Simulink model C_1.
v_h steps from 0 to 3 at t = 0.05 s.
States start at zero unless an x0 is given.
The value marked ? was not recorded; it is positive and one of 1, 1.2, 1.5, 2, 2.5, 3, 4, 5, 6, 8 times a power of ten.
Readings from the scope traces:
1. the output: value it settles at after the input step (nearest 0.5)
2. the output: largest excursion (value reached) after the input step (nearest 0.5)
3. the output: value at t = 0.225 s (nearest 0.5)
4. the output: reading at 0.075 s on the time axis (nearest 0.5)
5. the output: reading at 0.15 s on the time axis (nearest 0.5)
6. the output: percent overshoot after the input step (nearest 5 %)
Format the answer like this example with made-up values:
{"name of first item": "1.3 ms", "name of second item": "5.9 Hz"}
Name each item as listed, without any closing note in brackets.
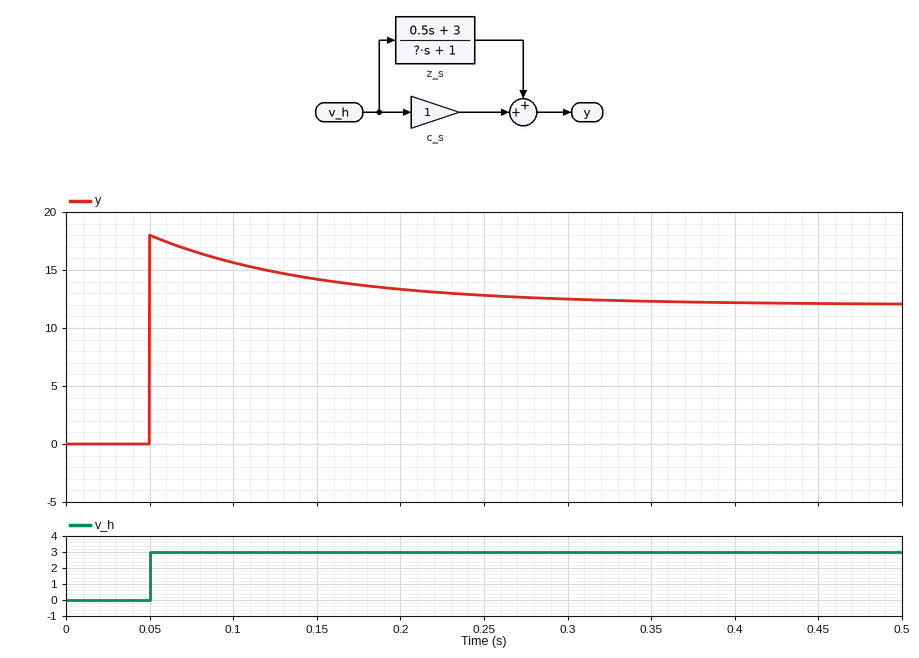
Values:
{"the output: value it settles at after the input step": "12.0", "the output: largest excursion (value reached) after the input step": "18.0", "the output: value at t = 0.225 s": "13.0", "the output: reading at 0.075 s on the time axis": "16.5", "the output: reading at 0.15 s on the time axis": "14.0", "the output: percent overshoot after the input step": "50 %"}
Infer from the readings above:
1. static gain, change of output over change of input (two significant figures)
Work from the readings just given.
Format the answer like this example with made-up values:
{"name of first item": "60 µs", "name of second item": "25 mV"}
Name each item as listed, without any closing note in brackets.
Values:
{"static gain, change of output over change of input": "4.0"}
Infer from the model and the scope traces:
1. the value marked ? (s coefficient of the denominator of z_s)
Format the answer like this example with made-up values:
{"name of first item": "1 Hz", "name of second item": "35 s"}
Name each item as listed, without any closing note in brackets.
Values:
{"the value marked ?": "0.1"}
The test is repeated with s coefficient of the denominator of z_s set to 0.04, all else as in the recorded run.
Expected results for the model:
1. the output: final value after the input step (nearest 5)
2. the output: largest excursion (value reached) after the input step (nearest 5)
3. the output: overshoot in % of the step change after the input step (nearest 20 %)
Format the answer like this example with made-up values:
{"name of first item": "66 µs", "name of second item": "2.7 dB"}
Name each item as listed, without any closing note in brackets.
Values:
{"the output: final value after the input step": "10", "the output: largest excursion (value reached) after the input step": "40", "the output: overshoot in % of the step change after the input step": "240 %"}
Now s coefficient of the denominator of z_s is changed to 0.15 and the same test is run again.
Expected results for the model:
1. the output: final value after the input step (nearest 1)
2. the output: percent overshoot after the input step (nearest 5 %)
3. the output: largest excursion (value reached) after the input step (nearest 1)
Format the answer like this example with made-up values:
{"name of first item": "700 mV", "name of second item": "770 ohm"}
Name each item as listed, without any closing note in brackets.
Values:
{"the output: final value after the input step": "12", "the output: percent overshoot after the input step": "10 %", "the output: largest excursion (value reached) after the input step": "13"}
